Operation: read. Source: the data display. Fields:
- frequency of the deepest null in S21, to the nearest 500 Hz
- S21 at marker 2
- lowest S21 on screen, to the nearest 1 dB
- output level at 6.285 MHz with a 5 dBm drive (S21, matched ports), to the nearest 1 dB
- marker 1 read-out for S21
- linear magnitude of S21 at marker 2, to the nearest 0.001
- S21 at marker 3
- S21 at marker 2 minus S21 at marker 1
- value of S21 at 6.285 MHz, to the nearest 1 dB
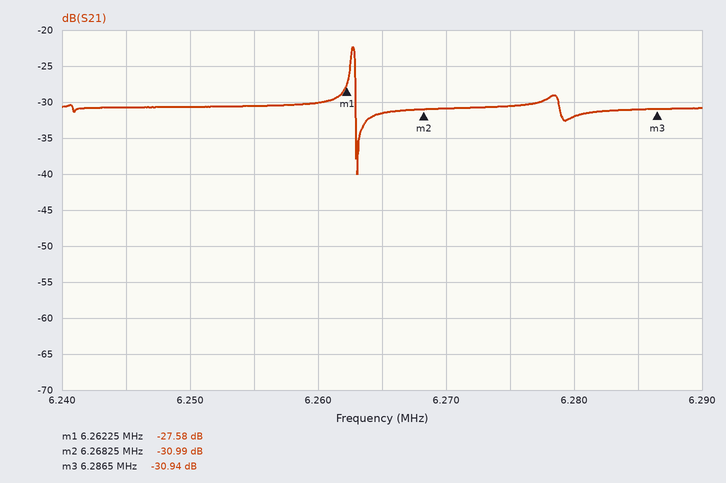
6.2630 MHz
-30.99 dB
-40 dB
-26 dBm
-27.58 dB
0.028
-30.94 dB
-3.41 dB
-31 dB
